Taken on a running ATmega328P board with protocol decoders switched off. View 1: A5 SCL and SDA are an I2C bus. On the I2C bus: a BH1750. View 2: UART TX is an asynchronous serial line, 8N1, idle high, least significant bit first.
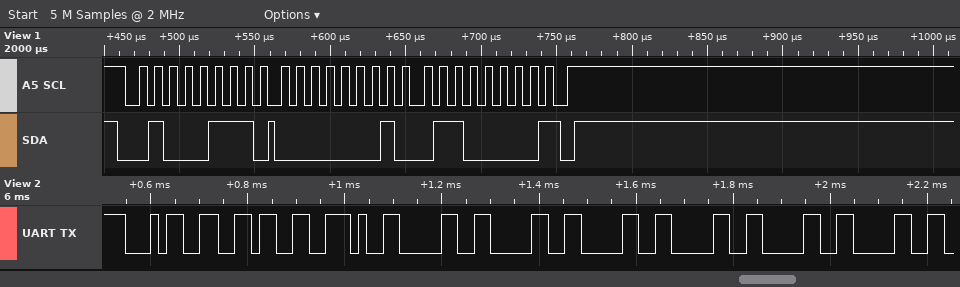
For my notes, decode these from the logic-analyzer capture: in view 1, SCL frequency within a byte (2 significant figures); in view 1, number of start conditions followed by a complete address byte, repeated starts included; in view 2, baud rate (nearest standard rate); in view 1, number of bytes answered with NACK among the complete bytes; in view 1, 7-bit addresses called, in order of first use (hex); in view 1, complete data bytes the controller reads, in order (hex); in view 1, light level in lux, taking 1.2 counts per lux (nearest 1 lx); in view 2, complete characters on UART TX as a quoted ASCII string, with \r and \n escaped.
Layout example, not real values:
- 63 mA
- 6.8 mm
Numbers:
- 100 kHz
- 1
- 57600 baud
- 1
- 0x23
- 01 60
- 293 lx
- "46.000000"
